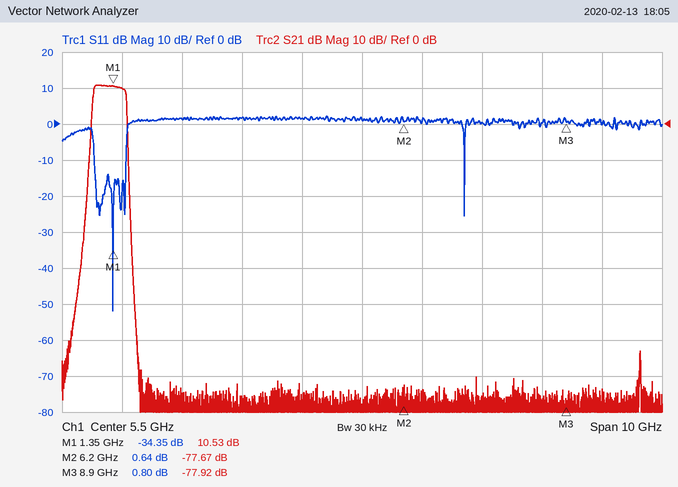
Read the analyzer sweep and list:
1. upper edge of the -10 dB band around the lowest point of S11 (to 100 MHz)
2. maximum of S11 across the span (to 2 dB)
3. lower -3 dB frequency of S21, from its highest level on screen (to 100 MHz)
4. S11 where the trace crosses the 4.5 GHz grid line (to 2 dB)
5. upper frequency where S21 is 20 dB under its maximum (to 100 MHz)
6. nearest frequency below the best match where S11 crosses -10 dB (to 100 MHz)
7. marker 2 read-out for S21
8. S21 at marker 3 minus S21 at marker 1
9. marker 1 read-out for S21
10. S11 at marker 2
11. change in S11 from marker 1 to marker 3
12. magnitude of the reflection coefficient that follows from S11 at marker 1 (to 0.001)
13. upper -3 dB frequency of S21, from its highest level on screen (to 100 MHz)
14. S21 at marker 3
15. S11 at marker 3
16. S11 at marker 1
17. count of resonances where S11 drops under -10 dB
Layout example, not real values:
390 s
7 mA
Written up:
1.6 GHz
2 dB
1.0 GHz
2 dB
1.6 GHz
1.0 GHz
-77.67 dB
-88.45 dB
10.53 dB
0.64 dB
35.15 dB
0.019
1.6 GHz
-77.92 dB
0.80 dB
-34.35 dB
5
